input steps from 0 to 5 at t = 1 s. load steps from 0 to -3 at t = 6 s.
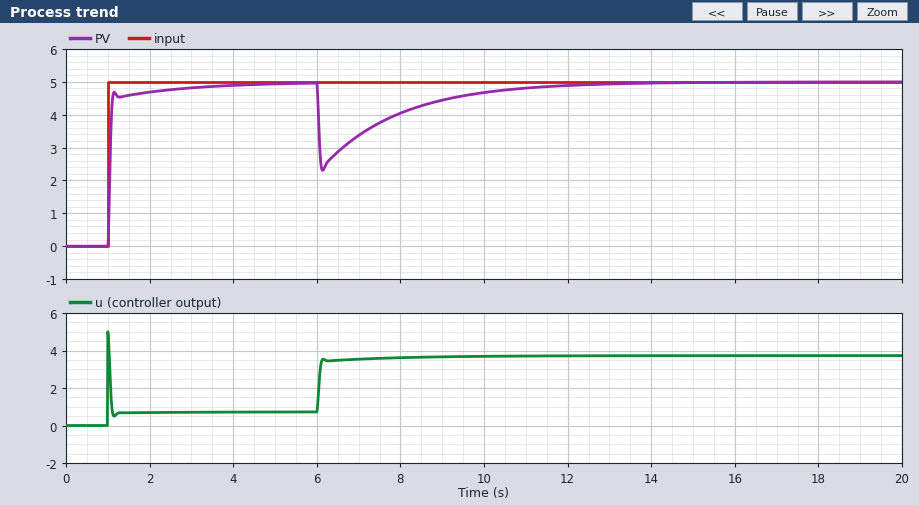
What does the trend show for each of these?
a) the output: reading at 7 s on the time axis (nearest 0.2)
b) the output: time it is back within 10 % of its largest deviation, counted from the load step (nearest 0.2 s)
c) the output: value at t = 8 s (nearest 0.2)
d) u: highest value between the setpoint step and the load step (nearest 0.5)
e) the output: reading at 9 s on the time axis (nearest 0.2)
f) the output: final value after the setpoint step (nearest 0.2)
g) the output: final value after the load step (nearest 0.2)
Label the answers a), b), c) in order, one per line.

a) 3.4
b) 4.4 s
c) 4.0
d) 5.0
e) 4.4
f) 5.0
g) 5.0
